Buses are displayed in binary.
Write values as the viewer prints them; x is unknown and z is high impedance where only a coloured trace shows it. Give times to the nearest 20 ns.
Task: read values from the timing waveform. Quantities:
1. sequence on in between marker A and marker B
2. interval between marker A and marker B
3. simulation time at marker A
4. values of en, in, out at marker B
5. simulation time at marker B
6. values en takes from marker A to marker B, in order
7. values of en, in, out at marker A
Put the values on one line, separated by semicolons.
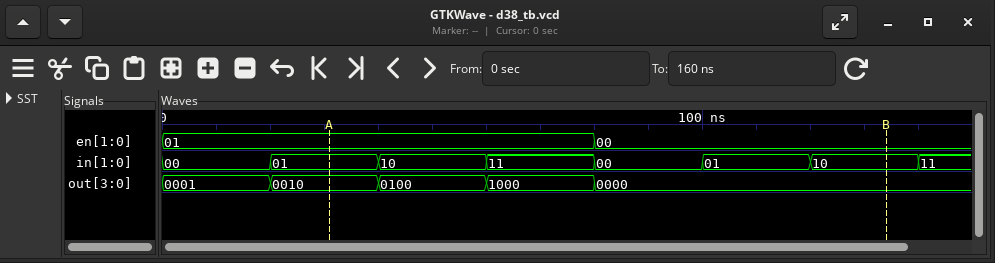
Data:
01, 10, 11, 00, 01, 10; 100 ns; 40 ns; en=00, in=10, out=0000; 140 ns; 01, 00; en=01, in=01, out=0010
